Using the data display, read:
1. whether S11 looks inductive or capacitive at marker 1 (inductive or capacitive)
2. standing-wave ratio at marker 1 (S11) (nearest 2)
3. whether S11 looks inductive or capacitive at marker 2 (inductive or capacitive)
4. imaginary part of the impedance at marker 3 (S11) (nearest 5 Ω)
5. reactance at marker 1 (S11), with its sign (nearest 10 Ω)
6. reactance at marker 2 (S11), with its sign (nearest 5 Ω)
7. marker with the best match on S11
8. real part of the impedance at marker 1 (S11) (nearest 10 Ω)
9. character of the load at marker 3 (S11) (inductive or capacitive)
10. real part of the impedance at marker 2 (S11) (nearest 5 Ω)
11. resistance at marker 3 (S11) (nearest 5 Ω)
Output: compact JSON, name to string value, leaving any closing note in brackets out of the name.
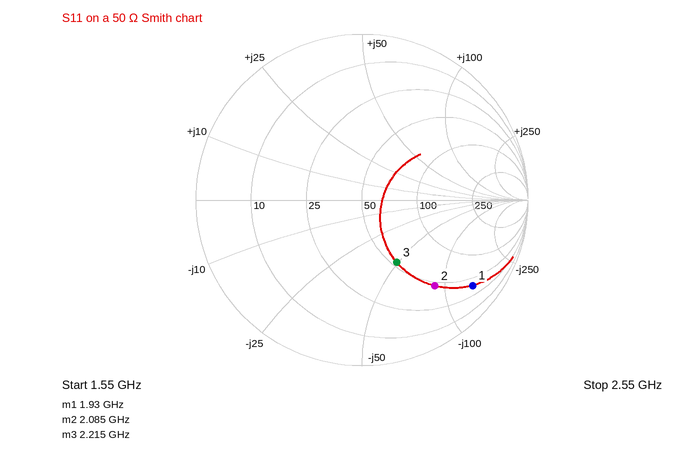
{"whether S11 looks inductive or capacitive at marker 1": "capacitive", "standing-wave ratio at marker 1 (S11)": "12", "whether S11 looks inductive or capacitive at marker 2": "capacitive", "imaginary part of the impedance at marker 3 (S11)": "-50 Ω", "reactance at marker 1 (S11), with its sign": "-140 Ω", "reactance at marker 2 (S11), with its sign": "-90 Ω", "marker with the best match on S11": "marker 3", "real part of the impedance at marker 1 (S11)": "40 Ω", "character of the load at marker 3 (S11)": "capacitive", "real part of the impedance at marker 2 (S11)": "45 Ω", "resistance at marker 3 (S11)": "55 Ω"}
